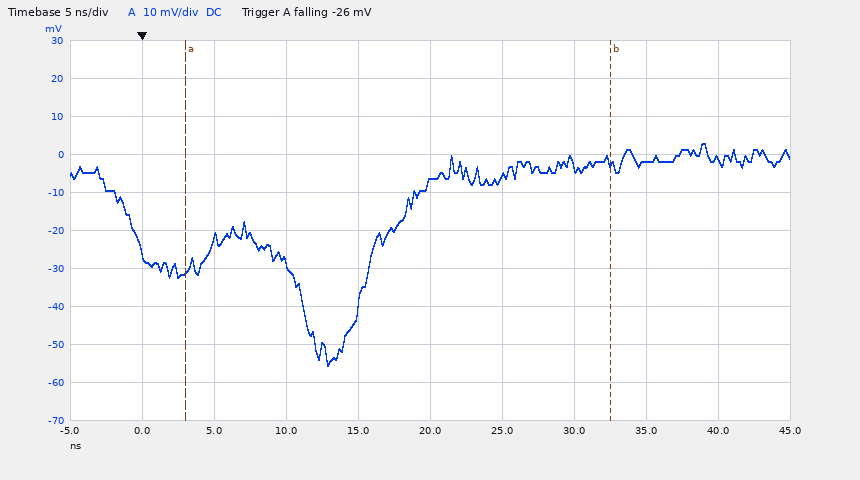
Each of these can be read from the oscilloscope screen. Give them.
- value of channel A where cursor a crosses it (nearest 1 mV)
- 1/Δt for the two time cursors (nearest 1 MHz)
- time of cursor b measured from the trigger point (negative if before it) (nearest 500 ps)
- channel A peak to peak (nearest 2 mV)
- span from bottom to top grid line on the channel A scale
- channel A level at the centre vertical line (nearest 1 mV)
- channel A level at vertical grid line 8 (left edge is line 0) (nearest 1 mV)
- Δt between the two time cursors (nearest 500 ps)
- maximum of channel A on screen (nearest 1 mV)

-31 mV
34 MHz
+32.5 ns
58 mV
100 mV
-7 mV
-2 mV
29.5 ns
3 mV
